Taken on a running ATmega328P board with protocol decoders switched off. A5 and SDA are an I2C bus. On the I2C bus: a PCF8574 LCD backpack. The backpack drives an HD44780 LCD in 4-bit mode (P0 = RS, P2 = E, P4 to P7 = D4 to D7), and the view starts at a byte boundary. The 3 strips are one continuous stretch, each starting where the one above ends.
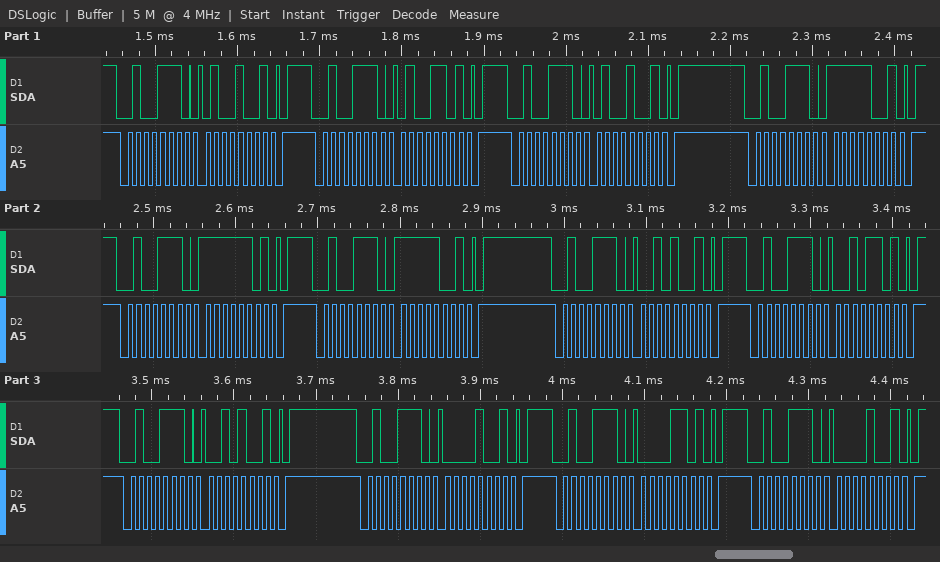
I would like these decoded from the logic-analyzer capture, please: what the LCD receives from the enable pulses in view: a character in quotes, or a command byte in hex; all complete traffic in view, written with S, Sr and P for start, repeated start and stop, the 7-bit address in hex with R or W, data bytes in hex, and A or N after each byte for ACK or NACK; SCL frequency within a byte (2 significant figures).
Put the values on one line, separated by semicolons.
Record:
'O' ' '; S 27W A 49 A P S 27W A 4D A P S 27W A 49 A P S 27W A F9 A P S 27W A FD A P S 27W A F9 A P S 27W A 29 A P S 27W A 2D A P S 27W A 29 A P S 27W A 09 A P S 27W A 0D A P S 27W A 09 A P; 100 kHz
